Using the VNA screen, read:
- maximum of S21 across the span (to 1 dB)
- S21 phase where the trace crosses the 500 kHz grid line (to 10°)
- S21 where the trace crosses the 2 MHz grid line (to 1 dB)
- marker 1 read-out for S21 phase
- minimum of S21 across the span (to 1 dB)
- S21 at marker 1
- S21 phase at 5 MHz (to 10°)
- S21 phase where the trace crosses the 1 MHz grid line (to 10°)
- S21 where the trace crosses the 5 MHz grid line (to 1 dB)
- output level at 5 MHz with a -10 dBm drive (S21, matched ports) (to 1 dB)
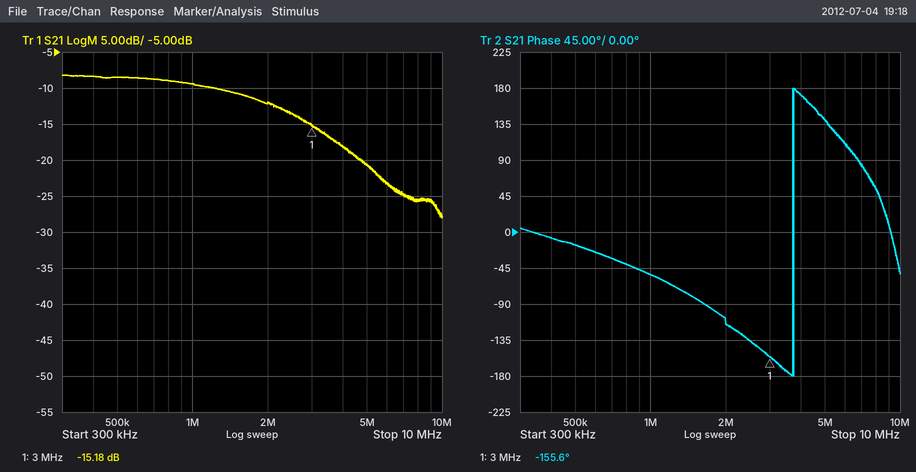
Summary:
-8 dB
-20°
-12 dB
-155.6°
-28 dB
-15.18 dB
140°
-50°
-21 dB
-31 dBm
